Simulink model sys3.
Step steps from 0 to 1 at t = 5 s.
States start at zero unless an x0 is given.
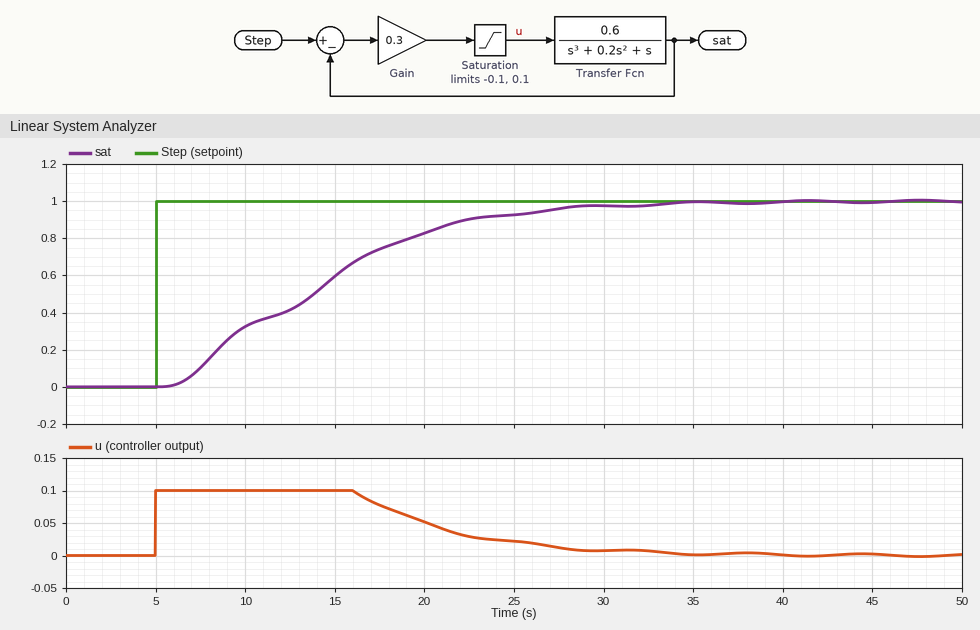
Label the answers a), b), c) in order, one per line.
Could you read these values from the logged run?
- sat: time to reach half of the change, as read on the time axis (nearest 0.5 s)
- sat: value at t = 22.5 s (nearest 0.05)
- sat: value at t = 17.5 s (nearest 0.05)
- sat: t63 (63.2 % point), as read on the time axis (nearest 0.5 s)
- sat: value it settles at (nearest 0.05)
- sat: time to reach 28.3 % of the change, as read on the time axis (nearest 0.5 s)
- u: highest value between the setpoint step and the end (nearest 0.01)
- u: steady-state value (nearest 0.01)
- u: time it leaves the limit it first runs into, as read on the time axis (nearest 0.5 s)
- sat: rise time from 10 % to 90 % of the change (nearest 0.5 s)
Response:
a) 14.0 s
b) 0.90
c) 0.75
d) 15.5 s
e) 1.00
f) 9.5 s
g) 0.10
h) 0.00
i) 16.0 s
j) 15.0 s
